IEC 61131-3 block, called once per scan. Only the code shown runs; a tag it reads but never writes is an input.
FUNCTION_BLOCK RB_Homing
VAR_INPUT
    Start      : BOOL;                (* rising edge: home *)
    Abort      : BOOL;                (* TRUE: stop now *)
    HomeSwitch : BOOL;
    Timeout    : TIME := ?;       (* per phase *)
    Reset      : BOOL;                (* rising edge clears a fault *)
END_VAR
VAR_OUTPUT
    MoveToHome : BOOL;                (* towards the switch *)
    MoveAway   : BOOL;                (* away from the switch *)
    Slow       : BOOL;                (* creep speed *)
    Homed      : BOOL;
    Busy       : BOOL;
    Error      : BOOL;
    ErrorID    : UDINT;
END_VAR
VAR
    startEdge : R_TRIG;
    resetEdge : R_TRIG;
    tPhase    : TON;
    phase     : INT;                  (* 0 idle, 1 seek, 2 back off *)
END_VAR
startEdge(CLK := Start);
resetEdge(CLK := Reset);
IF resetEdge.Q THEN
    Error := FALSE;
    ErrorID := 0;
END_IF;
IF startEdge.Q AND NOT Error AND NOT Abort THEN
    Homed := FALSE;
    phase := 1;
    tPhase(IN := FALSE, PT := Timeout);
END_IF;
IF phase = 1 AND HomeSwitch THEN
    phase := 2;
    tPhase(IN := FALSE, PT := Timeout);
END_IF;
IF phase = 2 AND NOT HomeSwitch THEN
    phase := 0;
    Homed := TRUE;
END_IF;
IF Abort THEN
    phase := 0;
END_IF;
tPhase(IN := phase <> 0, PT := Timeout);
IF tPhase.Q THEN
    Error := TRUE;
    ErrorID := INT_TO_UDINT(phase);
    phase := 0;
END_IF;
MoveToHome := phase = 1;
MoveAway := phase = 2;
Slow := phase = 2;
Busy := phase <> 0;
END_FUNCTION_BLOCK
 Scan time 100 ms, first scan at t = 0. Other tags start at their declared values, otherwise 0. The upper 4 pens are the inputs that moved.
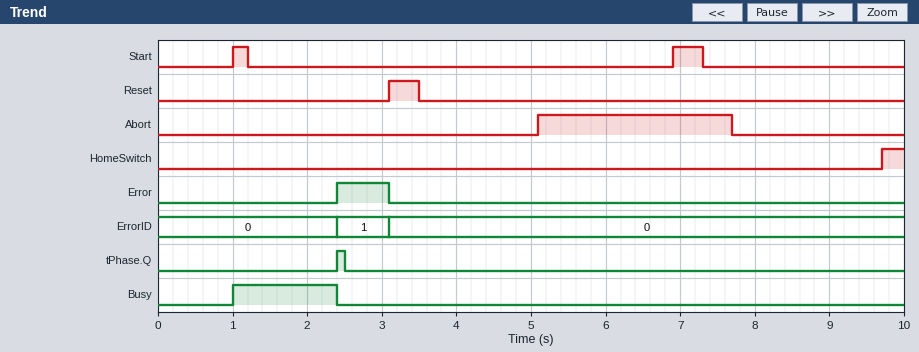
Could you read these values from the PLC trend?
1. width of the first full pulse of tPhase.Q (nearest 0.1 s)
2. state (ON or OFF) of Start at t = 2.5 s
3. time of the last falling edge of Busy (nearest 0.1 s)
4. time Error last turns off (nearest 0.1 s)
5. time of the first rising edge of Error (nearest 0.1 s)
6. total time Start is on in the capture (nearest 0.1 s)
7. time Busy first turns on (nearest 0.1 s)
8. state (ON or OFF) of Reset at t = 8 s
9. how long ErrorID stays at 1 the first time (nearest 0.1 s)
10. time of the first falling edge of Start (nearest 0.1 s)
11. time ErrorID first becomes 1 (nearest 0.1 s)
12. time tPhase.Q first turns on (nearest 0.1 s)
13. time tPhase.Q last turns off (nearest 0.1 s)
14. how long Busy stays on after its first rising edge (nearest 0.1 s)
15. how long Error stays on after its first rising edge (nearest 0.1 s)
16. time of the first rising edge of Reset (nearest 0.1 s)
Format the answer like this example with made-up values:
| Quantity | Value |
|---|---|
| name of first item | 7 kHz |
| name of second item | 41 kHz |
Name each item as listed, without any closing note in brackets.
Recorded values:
| Quantity | Value |
|---|---|
| width of the first full pulse of tPhase.Q | 0.1 s |
| state (ON or OFF) of Start at t = 2.5 s | OFF |
| time of the last falling edge of Busy | 2.4 s |
| time Error last turns off | 3.1 s |
| time of the first rising edge of Error | 2.4 s |
| total time Start is on in the capture | 0.6 s |
| time Busy first turns on | 1.0 s |
| state (ON or OFF) of Reset at t = 8 s | OFF |
| how long ErrorID stays at 1 the first time | 0.7 s |
| time of the first falling edge of Start | 1.2 s |
| time ErrorID first becomes 1 | 2.4 s |
| time tPhase.Q first turns on | 2.4 s |
| time tPhase.Q last turns off | 2.5 s |
| how long Busy stays on after its first rising edge | 1.4 s |
| how long Error stays on after its first rising edge | 0.7 s |
| time of the first rising edge of Reset | 3.1 s |
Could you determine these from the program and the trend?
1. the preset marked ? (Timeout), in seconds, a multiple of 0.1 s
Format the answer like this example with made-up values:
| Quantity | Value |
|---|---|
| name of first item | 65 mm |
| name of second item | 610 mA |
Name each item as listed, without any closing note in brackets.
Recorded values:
| Quantity | Value |
|---|---|
| the preset marked ? (Timeout), in seconds, a multiple of 0.1 s | 1.4 s |
